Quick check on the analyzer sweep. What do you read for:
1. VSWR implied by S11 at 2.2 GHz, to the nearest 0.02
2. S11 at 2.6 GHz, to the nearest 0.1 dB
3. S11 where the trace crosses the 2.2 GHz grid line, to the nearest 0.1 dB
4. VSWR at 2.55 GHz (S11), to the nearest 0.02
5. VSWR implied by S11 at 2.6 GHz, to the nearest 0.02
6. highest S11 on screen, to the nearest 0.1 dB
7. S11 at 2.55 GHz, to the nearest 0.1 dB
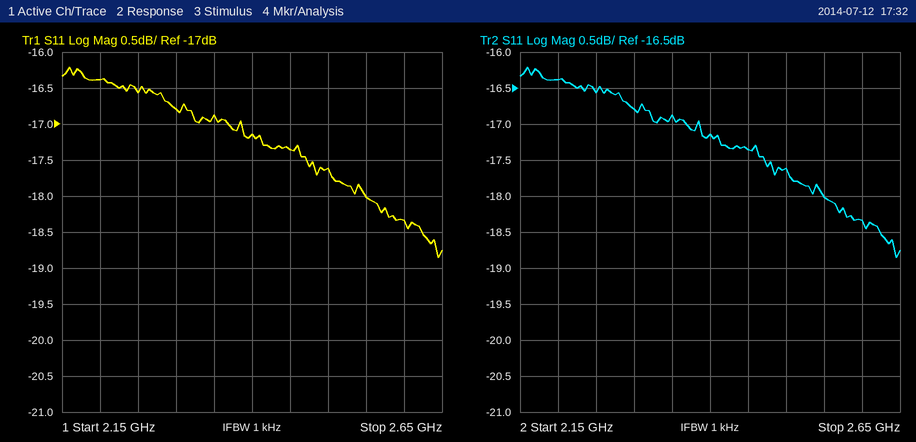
1.36
-18.3 dB
-16.4 dB
1.28
1.28
-16.2 dB
-18.0 dB
